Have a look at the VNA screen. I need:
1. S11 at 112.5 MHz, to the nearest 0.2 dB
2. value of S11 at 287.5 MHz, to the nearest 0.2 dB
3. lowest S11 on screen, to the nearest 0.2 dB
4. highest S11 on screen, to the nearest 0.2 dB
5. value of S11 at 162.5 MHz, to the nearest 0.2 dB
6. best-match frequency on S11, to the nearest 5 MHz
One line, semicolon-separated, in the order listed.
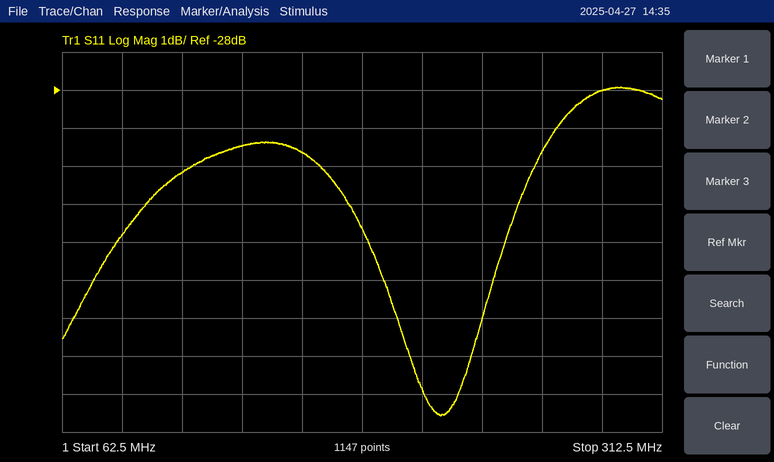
-30.2 dB; -28.0 dB; -36.6 dB; -28.0 dB; -29.6 dB; 220 MHz
